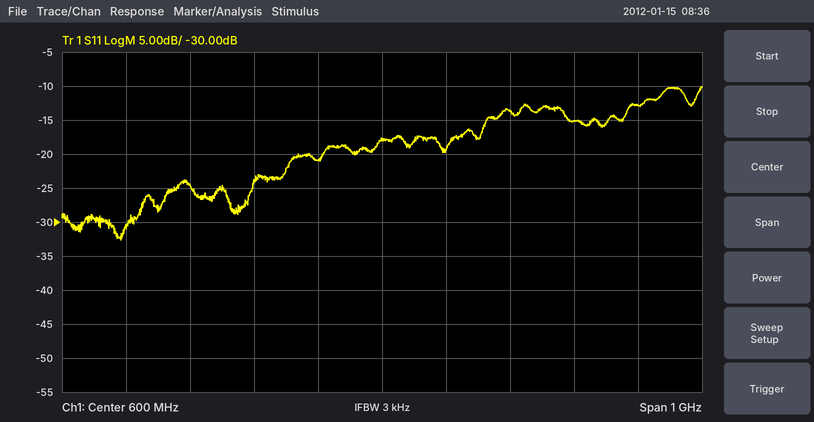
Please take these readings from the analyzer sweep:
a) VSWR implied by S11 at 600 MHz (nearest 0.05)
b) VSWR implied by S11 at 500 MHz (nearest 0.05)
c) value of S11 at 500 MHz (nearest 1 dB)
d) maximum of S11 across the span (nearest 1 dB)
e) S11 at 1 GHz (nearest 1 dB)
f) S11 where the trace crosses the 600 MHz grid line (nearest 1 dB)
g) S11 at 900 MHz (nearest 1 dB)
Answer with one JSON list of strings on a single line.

["1.30", "1.20", "-21 dB", "-10 dB", "-13 dB", "-18 dB", "-15 dB"]
